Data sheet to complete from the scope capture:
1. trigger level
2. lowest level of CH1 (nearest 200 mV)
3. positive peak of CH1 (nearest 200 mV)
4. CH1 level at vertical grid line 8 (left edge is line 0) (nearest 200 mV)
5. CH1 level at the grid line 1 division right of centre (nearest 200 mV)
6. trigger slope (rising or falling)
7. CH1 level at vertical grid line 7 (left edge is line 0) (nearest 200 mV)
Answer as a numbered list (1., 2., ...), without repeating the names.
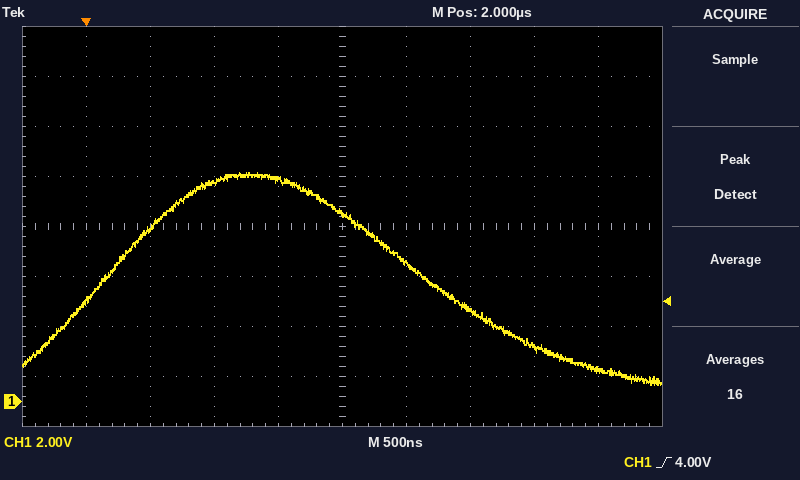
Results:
1. 4.00 V
2. 600 mV
3. 9.2 V
4. 2.2 V
5. 5.6 V
6. rising
7. 3.6 V
